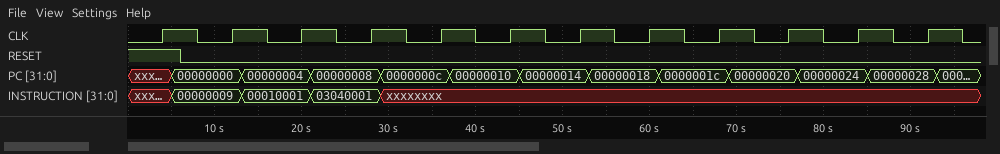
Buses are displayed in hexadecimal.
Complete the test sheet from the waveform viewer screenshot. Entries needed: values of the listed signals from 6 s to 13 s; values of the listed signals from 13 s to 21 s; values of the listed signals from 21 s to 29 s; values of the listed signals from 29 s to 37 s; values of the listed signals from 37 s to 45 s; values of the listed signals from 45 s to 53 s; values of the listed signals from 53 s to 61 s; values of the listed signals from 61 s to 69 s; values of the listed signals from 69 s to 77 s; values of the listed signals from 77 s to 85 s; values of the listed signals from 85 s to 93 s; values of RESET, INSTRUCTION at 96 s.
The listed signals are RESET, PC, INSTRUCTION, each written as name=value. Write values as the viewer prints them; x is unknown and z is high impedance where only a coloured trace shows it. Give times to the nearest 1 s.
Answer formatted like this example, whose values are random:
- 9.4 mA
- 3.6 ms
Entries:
- RESET=0, PC=00000000, INSTRUCTION=00000009
- RESET=0, PC=00000004, INSTRUCTION=00010001
- RESET=0, PC=00000008, INSTRUCTION=03040001
- RESET=0, PC=0000000c, INSTRUCTION=xxxxxxxx
- RESET=0, PC=00000010, INSTRUCTION=xxxxxxxx
- RESET=0, PC=00000014, INSTRUCTION=xxxxxxxx
- RESET=0, PC=00000018, INSTRUCTION=xxxxxxxx
- RESET=0, PC=0000001c, INSTRUCTION=xxxxxxxx
- RESET=0, PC=00000020, INSTRUCTION=xxxxxxxx
- RESET=0, PC=00000024, INSTRUCTION=xxxxxxxx
- RESET=0, PC=00000028, INSTRUCTION=xxxxxxxx
- RESET=0, INSTRUCTION=xxxxxxxx
